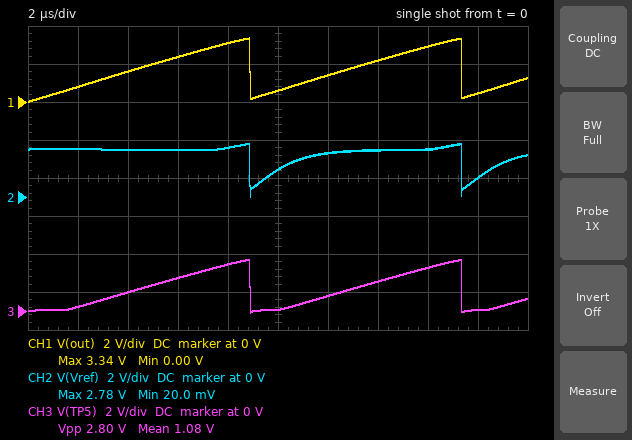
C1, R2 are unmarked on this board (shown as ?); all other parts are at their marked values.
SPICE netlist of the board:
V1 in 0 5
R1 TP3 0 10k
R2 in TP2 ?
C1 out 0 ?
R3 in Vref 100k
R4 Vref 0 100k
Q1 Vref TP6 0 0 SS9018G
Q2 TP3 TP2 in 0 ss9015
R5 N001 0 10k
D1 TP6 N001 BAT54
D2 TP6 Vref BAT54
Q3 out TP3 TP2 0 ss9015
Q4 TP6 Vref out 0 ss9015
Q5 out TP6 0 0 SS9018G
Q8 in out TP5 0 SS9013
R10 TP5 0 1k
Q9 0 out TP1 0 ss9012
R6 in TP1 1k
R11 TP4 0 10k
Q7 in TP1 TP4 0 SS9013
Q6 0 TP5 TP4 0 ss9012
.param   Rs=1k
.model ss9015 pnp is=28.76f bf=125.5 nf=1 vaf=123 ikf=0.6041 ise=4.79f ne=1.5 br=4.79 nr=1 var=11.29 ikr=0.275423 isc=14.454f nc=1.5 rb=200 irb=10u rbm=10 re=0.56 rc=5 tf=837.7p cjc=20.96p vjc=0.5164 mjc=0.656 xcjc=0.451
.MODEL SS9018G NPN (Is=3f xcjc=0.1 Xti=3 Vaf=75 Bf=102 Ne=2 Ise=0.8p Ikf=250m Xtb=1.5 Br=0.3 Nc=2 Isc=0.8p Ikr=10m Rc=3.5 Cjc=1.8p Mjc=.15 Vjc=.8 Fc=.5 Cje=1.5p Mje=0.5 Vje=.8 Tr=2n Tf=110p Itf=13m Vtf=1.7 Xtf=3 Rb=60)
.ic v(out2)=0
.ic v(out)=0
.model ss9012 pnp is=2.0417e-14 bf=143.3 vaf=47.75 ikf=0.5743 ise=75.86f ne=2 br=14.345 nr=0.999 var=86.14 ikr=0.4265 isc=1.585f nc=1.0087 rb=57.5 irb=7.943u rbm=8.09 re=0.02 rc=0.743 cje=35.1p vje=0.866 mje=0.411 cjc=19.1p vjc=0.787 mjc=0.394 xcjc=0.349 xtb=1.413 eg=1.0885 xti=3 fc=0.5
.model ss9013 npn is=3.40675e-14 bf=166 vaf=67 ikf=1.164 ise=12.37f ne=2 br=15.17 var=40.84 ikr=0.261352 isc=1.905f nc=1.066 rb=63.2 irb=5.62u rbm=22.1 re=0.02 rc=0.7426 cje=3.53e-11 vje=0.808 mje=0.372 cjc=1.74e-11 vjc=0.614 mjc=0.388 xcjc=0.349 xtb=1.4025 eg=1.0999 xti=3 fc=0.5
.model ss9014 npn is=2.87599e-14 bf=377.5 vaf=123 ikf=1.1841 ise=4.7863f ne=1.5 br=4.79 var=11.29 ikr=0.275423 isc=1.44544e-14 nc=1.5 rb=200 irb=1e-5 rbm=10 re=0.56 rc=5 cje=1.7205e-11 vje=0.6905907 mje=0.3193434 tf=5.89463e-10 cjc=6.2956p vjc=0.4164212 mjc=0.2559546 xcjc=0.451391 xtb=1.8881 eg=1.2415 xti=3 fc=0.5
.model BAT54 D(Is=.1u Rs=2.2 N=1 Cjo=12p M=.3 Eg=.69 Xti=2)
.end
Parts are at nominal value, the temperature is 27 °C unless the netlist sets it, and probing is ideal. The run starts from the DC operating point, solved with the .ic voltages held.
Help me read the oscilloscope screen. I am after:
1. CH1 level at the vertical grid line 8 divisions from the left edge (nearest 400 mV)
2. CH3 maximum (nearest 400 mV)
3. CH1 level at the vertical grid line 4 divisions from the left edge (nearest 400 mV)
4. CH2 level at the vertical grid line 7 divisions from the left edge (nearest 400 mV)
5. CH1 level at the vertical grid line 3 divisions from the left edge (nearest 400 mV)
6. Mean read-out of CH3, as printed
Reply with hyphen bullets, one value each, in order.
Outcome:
- 2.8 V
- 2.8 V
- 3.2 V
- 2.4 V
- 2.4 V
- 1.08 V
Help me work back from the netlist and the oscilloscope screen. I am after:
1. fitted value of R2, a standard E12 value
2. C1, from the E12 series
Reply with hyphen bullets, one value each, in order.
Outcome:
- 3.3 kΩ
- 470 pF
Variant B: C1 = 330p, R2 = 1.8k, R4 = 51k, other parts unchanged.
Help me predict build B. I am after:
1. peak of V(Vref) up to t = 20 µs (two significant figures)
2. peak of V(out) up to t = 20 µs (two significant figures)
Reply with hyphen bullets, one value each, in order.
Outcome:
- 2.0 V
- 2.6 V
